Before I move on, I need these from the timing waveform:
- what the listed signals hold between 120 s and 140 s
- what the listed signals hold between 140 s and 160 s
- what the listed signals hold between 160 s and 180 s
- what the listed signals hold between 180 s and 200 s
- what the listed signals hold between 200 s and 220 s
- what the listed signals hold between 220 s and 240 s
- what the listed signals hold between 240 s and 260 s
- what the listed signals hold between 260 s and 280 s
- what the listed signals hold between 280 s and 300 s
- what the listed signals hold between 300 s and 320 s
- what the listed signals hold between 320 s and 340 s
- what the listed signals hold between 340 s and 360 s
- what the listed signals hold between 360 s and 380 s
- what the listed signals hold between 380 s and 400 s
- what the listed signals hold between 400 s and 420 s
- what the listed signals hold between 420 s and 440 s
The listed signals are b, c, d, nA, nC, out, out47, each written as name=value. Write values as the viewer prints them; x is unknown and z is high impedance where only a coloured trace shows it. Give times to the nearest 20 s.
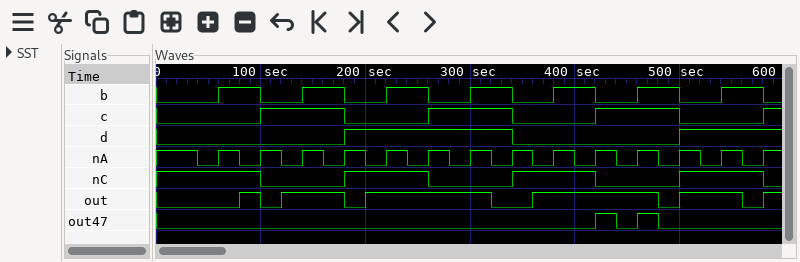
b=0, c=1, d=0, nA=0, nC=0, out=1, out47=0
b=1, c=1, d=0, nA=1, nC=0, out=1, out47=0
b=1, c=1, d=0, nA=0, nC=0, out=1, out47=0
b=0, c=0, d=1, nA=1, nC=1, out=0, out47=0
b=0, c=0, d=1, nA=0, nC=1, out=1, out47=0
b=1, c=0, d=1, nA=1, nC=1, out=1, out47=0
b=1, c=0, d=1, nA=0, nC=1, out=1, out47=0
b=0, c=1, d=1, nA=1, nC=0, out=1, out47=0
b=0, c=1, d=1, nA=0, nC=0, out=1, out47=0
b=1, c=1, d=1, nA=1, nC=0, out=1, out47=0
b=1, c=1, d=1, nA=0, nC=0, out=0, out47=0
b=0, c=0, d=0, nA=1, nC=1, out=0, out47=0
b=0, c=0, d=0, nA=0, nC=1, out=1, out47=0
b=1, c=0, d=0, nA=1, nC=1, out=1, out47=0
b=1, c=0, d=0, nA=0, nC=1, out=1, out47=0
b=0, c=1, d=0, nA=1, nC=0, out=1, out47=1
